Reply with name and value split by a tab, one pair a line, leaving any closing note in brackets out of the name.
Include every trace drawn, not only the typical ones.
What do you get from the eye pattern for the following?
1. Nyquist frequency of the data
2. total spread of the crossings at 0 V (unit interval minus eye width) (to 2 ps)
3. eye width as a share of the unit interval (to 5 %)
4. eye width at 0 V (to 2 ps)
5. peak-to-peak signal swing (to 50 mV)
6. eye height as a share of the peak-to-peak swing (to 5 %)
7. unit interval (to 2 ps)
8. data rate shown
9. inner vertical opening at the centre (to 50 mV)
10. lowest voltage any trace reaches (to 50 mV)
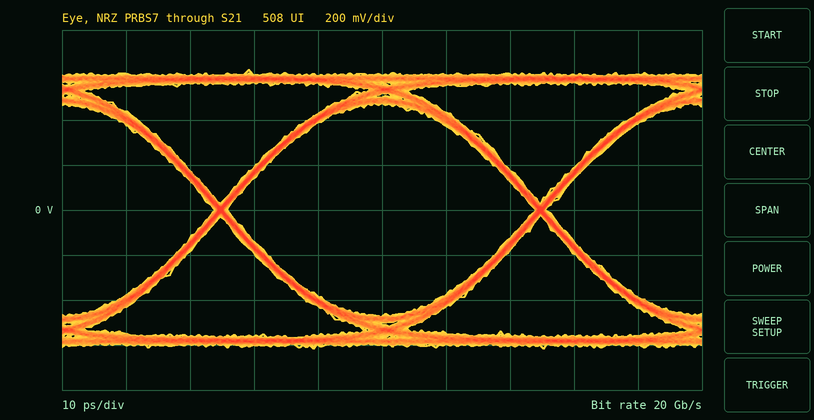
Nyquist frequency of the data	10 GHz
total spread of the crossings at 0 V (unit interval minus eye width)	2 ps
eye width as a share of the unit interval	95 %
eye width at 0 V	48 ps
peak-to-peak signal swing	1.25 V
eye height as a share of the peak-to-peak swing	75 %
unit interval	50 ps
data rate shown	20 Gb/s
inner vertical opening at the centre	950 mV
lowest voltage any trace reaches	-600 mV
